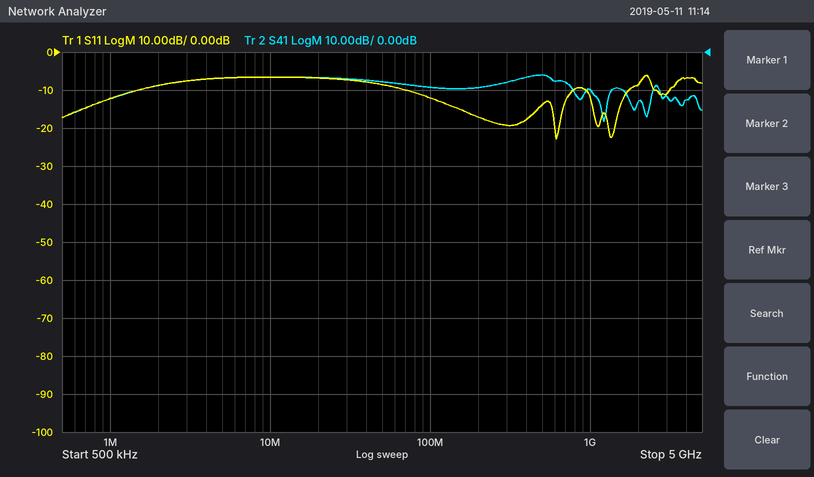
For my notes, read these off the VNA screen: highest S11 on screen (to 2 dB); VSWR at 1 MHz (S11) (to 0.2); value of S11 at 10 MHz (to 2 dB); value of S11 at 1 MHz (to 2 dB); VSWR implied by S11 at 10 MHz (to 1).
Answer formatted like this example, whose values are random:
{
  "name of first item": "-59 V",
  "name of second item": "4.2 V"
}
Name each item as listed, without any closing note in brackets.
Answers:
{
  "highest S11 on screen": "-6 dB",
  "VSWR at 1 MHz (S11)": "1.6",
  "value of S11 at 10 MHz": "-6 dB",
  "value of S11 at 1 MHz": "-12 dB",
  "VSWR implied by S11 at 10 MHz": "3"
}
